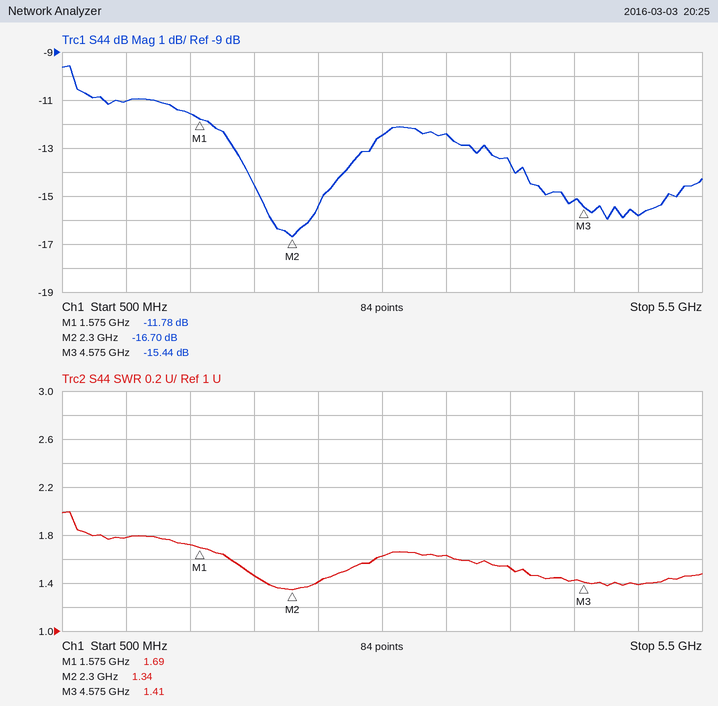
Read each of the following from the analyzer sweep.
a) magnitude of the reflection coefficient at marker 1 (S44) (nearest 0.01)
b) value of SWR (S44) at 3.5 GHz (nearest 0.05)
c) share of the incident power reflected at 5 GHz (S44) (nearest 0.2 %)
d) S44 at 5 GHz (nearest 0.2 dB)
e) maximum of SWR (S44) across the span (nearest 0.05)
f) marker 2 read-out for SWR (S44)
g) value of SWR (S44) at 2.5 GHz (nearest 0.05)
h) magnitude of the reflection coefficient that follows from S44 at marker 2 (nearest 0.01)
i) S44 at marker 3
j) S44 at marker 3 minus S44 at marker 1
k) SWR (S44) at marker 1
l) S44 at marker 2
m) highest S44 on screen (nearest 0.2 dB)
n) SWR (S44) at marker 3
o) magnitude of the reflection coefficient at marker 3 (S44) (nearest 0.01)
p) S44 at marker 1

0.26
1.65
2.6 %
-15.8 dB
2.00
1.34
1.40
0.15
-15.44 dB
-3.66 dB
1.69
-16.70 dB
-9.6 dB
1.41
0.17
-11.78 dB
